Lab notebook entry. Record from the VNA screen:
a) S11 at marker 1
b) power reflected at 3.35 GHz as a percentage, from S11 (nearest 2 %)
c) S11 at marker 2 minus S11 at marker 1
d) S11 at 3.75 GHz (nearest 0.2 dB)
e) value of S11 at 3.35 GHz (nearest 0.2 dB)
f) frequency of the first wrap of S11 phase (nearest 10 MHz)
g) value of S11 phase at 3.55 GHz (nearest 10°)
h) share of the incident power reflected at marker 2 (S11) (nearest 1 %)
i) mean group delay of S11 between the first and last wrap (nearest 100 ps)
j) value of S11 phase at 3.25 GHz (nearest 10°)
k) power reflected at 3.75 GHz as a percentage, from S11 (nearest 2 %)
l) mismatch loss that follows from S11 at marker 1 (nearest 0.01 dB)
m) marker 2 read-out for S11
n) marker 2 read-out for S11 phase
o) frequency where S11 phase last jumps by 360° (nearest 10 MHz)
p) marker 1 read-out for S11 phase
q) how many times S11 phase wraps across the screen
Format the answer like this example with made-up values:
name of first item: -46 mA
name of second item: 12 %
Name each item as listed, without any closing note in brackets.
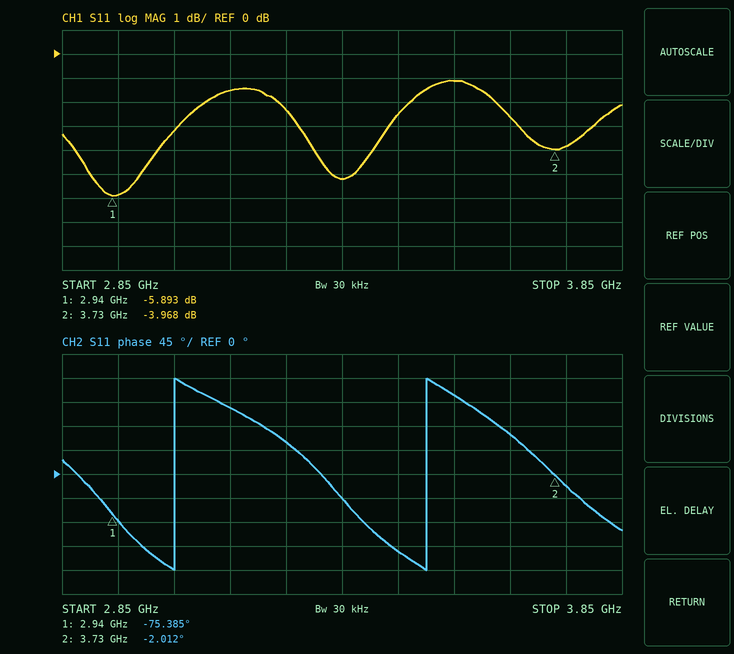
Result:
S11 at marker 1: -5.893 dB
power reflected at 3.35 GHz as a percentage, from S11: 30 %
S11 at marker 2 minus S11 at marker 1: 1.925 dB
S11 at 3.75 GHz: -3.8 dB
value of S11 at 3.35 GHz: -5.2 dB
frequency of the first wrap of S11 phase: 3.05 GHz
value of S11 phase at 3.55 GHz: 150°
share of the incident power reflected at marker 2 (S11): 40 %
mean group delay of S11 between the first and last wrap: 2.2 ns
value of S11 phase at 3.25 GHz: 60°
power reflected at 3.75 GHz as a percentage, from S11: 42 %
mismatch loss that follows from S11 at marker 1: 1.29 dB
marker 2 read-out for S11: -3.968 dB
marker 2 read-out for S11 phase: -2.012°
frequency where S11 phase last jumps by 360°: 3.50 GHz
marker 1 read-out for S11 phase: -75.385°
how many times S11 phase wraps across the screen: 2
